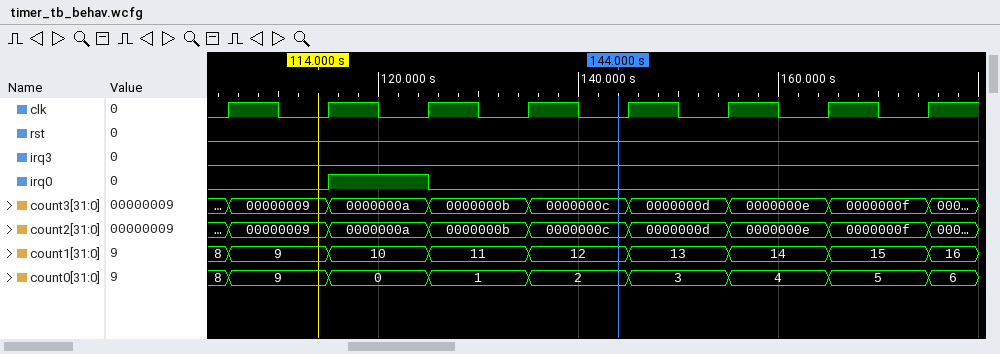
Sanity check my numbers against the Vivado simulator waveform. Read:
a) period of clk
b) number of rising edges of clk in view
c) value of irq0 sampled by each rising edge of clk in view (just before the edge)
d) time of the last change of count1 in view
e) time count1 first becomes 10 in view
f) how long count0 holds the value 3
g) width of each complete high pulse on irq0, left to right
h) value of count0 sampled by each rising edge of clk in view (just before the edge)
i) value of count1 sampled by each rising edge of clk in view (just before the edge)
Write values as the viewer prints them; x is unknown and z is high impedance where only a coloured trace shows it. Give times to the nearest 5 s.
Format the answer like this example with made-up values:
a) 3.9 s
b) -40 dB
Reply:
a) 10 s
b) 8
c) 0 0 1 0 0 0 0 0
d) 175 s
e) 115 s
f) 10 s
g) 10 s
h) 8, 9, 0, 1, 2, 3, 4, 5
i) 8, 9, 10, 11, 12, 13, 14, 15
